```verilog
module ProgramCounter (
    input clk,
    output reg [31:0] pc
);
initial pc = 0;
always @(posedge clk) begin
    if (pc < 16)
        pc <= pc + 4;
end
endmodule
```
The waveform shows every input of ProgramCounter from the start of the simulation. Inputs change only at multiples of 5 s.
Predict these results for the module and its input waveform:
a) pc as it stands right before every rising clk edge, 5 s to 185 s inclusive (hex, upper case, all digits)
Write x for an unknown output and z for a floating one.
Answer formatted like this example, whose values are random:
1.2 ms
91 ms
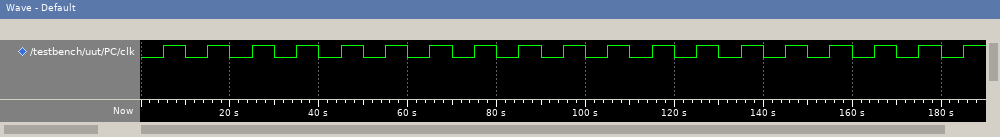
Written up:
00000000, 00000004, 00000008, 0000000C, 00000010, 00000010, 00000010, 00000010, 00000010, 00000010, 00000010, 00000010, 00000010, 00000010, 00000010, 00000010, 00000010, 00000010, 00000010
